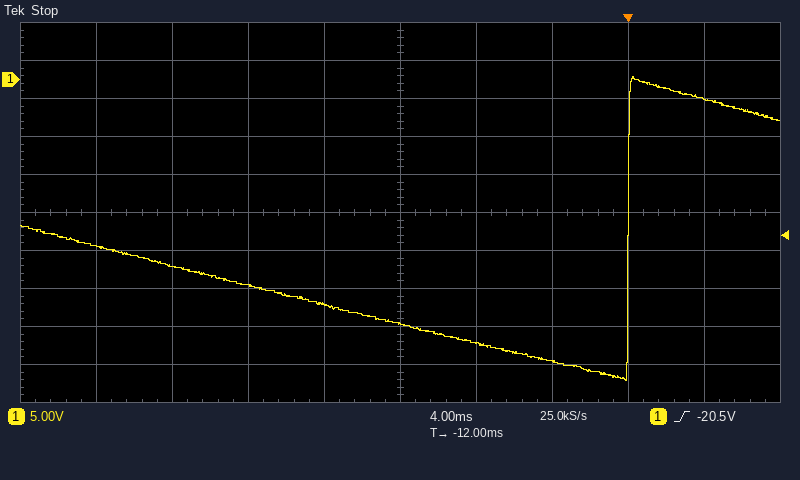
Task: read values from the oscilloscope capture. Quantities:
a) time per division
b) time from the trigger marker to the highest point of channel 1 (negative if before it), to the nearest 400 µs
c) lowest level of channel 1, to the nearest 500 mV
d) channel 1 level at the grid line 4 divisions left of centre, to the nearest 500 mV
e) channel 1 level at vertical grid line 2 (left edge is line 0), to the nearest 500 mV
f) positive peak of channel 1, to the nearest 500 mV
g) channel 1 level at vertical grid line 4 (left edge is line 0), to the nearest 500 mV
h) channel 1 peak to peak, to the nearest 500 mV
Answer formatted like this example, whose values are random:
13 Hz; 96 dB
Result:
4 ms; +400 µs; -39.5 V; -22.0 V; -24.5 V; 500 mV; -29.5 V; 40.0 V
